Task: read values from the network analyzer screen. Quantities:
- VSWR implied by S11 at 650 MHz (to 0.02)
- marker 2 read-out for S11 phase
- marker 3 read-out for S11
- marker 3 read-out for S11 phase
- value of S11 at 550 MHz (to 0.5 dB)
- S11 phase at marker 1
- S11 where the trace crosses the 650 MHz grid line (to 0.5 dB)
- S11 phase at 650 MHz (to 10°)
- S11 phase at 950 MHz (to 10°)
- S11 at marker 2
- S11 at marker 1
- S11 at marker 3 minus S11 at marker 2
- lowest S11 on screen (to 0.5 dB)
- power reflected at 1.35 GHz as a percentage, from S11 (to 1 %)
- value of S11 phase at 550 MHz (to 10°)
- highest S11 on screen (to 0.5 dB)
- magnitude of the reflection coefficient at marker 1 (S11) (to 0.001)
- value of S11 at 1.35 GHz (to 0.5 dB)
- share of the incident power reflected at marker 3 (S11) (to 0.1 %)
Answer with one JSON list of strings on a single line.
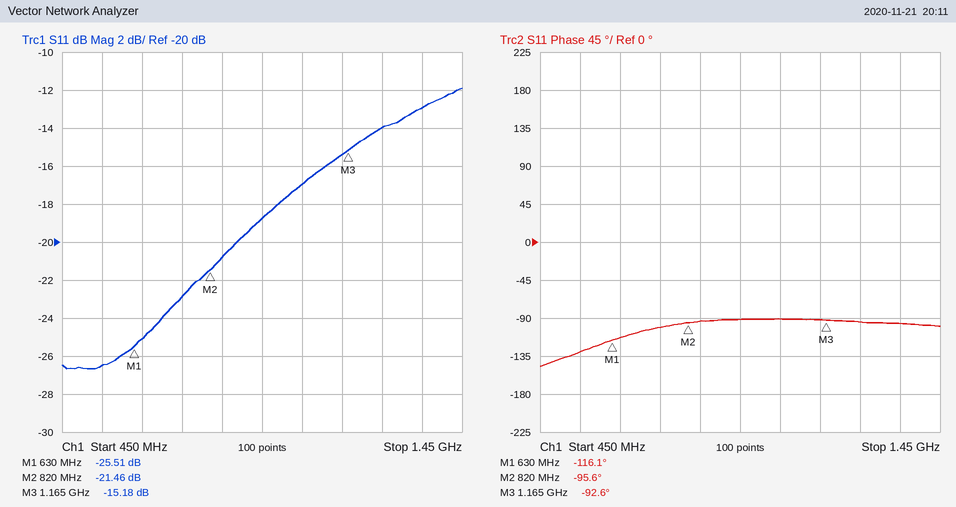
["1.12", "-95.6°", "-15.18 dB", "-92.6°", "-26.5 dB", "-116.1°", "-25.0 dB", "-110°", "-90°", "-21.46 dB", "-25.51 dB", "6.28 dB", "-26.5 dB", "5 %", "-130°", "-12.0 dB", "0.053", "-13.0 dB", "3.0 %"]
